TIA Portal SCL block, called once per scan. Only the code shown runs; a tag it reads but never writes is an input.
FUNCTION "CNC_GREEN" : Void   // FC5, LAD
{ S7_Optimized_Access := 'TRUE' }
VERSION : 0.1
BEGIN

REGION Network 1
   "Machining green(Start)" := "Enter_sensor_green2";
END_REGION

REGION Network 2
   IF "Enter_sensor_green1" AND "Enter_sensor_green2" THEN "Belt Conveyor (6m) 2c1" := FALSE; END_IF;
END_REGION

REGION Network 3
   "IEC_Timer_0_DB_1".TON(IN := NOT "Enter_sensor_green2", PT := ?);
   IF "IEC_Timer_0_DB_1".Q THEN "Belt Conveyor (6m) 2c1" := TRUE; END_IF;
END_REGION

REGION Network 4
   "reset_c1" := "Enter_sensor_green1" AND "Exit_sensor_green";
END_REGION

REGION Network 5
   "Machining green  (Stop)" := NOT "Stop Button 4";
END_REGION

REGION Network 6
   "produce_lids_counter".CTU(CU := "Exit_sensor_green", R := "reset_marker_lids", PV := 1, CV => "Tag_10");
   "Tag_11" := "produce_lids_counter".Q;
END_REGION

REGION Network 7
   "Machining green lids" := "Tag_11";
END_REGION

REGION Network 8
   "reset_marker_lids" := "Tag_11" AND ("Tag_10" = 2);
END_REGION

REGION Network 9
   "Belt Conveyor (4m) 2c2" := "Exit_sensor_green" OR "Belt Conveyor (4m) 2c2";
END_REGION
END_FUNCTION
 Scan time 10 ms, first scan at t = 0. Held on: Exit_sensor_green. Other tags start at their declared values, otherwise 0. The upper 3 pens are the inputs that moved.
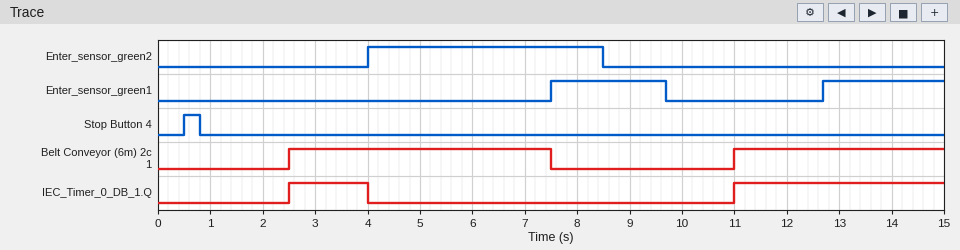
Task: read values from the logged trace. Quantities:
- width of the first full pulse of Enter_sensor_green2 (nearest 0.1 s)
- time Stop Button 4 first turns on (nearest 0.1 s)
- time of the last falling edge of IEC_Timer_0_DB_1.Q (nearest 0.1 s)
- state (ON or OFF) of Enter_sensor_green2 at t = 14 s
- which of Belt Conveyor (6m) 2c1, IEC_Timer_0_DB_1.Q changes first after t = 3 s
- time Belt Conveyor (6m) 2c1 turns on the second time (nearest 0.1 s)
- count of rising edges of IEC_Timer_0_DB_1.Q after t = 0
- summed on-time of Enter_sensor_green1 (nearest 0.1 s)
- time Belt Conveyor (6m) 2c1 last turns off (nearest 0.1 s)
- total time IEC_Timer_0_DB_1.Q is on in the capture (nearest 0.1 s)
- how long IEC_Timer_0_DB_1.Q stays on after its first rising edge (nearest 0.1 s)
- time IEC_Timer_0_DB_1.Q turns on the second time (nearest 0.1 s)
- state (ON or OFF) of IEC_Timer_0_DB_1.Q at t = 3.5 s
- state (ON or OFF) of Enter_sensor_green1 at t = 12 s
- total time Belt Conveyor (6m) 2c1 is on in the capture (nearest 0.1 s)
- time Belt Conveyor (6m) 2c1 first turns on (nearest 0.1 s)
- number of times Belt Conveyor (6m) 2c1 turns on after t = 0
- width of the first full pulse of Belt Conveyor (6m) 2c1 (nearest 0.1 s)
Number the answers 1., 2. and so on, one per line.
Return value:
1. 4.5 s
2. 0.5 s
3. 4.0 s
4. OFF
5. IEC_Timer_0_DB_1.Q
6. 11.0 s
7. 2
8. 4.5 s
9. 7.5 s
10. 5.5 s
11. 1.5 s
12. 11.0 s
13. ON
14. OFF
15. 9.0 s
16. 2.5 s
17. 2
18. 5.0 s
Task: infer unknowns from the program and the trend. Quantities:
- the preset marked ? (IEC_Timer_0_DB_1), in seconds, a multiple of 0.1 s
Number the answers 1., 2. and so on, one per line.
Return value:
1. 2.5 s
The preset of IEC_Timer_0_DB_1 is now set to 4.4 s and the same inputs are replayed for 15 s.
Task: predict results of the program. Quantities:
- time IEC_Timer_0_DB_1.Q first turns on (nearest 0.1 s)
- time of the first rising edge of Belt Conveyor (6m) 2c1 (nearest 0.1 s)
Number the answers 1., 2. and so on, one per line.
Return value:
1. 12.9 s
2. 12.9 s
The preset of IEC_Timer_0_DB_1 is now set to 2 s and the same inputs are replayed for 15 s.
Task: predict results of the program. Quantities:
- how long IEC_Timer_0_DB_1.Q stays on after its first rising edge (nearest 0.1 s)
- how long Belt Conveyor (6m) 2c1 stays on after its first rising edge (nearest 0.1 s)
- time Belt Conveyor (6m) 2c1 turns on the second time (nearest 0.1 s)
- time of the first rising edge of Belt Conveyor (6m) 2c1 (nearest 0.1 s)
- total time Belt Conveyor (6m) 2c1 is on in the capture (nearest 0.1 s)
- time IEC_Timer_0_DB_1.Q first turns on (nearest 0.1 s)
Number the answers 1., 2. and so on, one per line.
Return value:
1. 2.0 s
2. 5.5 s
3. 10.5 s
4. 2.0 s
5. 10.0 s
6. 2.0 s
